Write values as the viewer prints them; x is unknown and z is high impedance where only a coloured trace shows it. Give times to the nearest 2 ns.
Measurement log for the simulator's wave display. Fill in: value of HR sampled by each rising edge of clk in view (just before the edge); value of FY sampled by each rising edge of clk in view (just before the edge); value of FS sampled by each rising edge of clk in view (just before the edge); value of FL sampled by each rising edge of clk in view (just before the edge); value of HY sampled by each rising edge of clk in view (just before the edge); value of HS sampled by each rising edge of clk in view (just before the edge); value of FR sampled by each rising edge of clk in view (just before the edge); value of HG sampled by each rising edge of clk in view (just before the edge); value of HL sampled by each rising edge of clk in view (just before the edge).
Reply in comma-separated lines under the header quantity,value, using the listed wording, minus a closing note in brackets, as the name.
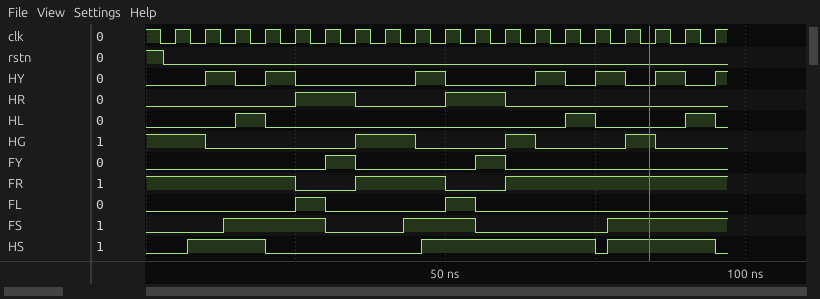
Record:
quantity,value
value of HR sampled by each rising edge of clk in view,0 0 0 0 0 1 1 0 0 0 1 1 0 0 0 0 0 0 0
value of FY sampled by each rising edge of clk in view,0 0 0 0 0 0 1 0 0 0 0 1 0 0 0 0 0 0 0
value of FS sampled by each rising edge of clk in view,0 0 1 1 1 1 0 0 1 1 1 0 0 0 0 1 1 1 1
value of FL sampled by each rising edge of clk in view,0 0 0 0 0 1 0 0 0 0 1 0 0 0 0 0 0 0 0
value of HY sampled by each rising edge of clk in view,0 0 1 0 1 0 0 0 0 1 0 0 0 1 0 1 0 1 0
value of HS sampled by each rising edge of clk in view,0 1 1 1 0 0 0 0 0 1 1 1 1 1 1 1 1 1 1
value of FR sampled by each rising edge of clk in view,1 1 1 1 1 0 0 1 1 1 0 0 1 1 1 1 1 1 1
value of HG sampled by each rising edge of clk in view,1 1 0 0 0 0 0 1 1 0 0 0 1 0 0 0 1 0 0
value of HL sampled by each rising edge of clk in view,0 0 0 1 0 0 0 0 0 0 0 0 0 0 1 0 0 0 1
